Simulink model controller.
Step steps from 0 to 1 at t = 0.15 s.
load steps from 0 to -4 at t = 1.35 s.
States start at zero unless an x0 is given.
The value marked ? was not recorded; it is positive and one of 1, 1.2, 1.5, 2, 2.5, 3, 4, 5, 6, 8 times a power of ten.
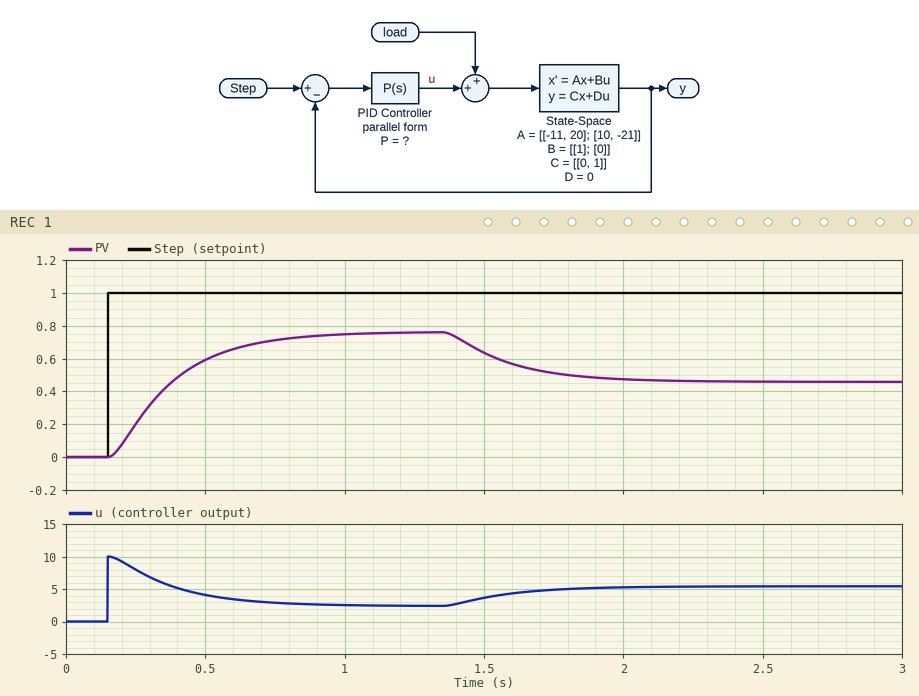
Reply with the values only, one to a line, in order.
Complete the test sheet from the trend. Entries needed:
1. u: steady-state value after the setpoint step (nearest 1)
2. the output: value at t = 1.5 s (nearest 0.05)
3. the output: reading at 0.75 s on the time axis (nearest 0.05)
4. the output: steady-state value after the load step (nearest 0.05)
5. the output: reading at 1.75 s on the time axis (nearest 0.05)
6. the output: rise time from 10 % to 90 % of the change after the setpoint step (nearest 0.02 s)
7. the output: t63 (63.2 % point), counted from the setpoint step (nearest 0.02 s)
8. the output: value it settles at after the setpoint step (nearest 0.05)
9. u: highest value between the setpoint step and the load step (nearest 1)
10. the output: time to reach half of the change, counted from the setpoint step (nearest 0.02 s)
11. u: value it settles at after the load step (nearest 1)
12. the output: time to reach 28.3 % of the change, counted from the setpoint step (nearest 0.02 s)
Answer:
2
0.65
0.70
0.45
0.50
0.46 s
0.24 s
0.75
10
0.18 s
5
0.10 s
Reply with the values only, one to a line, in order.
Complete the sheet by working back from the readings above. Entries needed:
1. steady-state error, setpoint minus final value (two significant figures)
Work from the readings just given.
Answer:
0.25
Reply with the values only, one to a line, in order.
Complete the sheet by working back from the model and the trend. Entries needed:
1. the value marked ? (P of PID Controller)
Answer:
10
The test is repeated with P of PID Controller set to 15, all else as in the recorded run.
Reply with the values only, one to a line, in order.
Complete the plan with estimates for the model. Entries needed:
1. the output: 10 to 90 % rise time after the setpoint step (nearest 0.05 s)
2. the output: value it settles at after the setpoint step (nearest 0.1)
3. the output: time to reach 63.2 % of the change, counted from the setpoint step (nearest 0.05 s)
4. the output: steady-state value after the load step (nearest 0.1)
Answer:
0.30 s
0.8
0.20 s
0.6
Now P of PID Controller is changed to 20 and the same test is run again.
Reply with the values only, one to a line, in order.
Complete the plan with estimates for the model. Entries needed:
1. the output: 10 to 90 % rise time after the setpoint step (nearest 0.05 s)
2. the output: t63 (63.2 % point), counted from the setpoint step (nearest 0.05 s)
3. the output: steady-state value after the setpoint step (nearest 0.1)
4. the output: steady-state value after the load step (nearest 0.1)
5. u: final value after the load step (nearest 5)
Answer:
0.25 s
0.15 s
0.9
0.7
5
